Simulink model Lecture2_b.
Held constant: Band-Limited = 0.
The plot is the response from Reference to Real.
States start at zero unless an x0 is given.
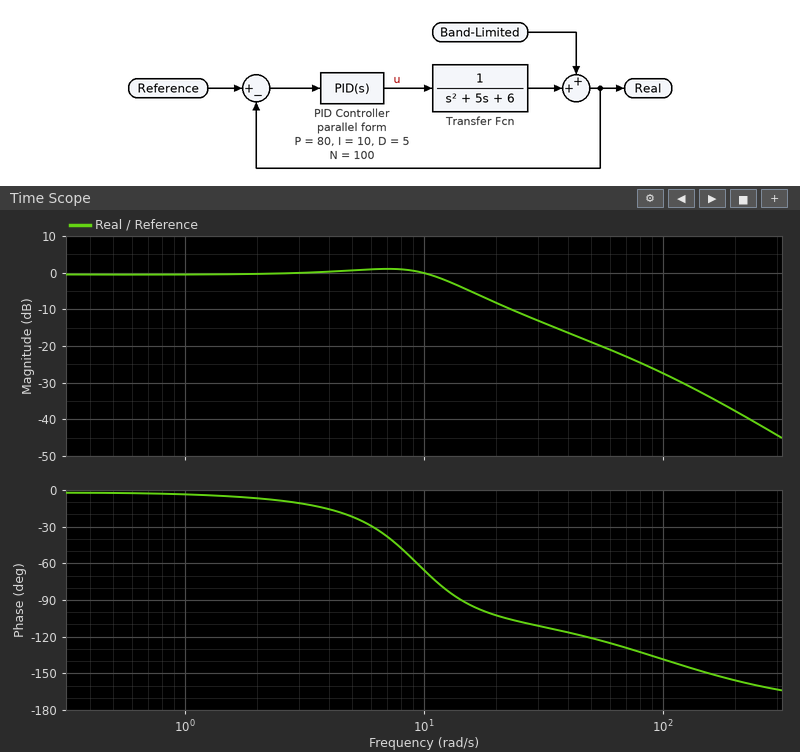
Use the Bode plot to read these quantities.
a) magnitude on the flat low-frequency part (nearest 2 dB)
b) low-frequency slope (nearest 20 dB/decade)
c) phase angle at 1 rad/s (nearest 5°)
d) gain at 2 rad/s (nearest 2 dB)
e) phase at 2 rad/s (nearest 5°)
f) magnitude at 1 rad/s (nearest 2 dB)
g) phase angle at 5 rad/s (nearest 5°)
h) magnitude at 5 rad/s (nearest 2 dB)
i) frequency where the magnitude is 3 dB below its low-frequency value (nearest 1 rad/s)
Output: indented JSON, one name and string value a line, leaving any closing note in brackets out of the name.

{
  "magnitude on the flat low-frequency part": "0 dB",
  "low-frequency slope": "0 dB/decade",
  "phase angle at 1 rad/s": "-5°",
  "gain at 2 rad/s": "0 dB",
  "phase at 2 rad/s": "-5°",
  "magnitude at 1 rad/s": "0 dB",
  "phase angle at 5 rad/s": "-20°",
  "magnitude at 5 rad/s": "0 dB",
  "frequency where the magnitude is 3 dB below its low-frequency value": "14 rad/s"
}
